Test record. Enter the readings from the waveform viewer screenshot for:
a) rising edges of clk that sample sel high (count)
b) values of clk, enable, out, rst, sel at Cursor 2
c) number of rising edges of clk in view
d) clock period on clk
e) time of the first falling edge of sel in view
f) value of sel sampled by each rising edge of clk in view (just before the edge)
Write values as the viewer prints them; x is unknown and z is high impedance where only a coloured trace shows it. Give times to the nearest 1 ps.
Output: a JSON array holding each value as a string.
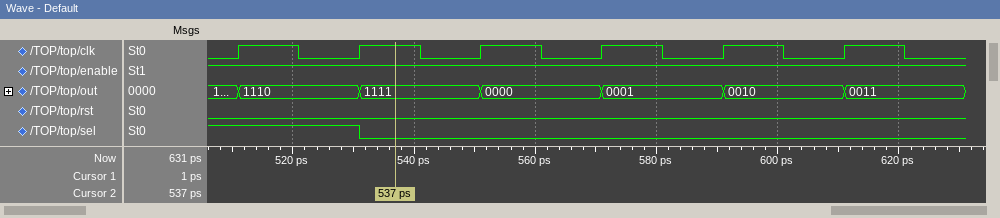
["2", "clk=1, enable=1, out=1111, rst=0, sel=0", "6", "20 ps", "531 ps", "1 1 0 0 0 0"]
